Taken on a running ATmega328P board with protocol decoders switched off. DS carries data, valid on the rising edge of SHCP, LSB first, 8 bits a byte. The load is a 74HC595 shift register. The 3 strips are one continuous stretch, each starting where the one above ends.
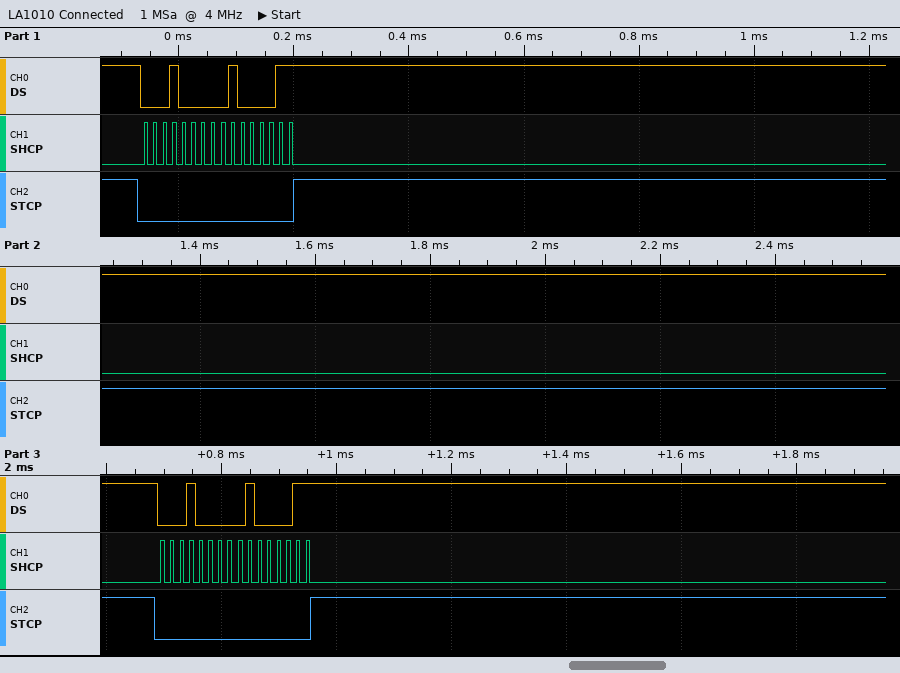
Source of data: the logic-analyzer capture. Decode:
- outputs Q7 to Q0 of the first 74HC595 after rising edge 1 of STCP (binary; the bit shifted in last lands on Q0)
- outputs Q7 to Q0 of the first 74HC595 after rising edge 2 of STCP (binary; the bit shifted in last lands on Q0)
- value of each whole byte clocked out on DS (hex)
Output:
01000011
01000011
08 C2 08 C2
